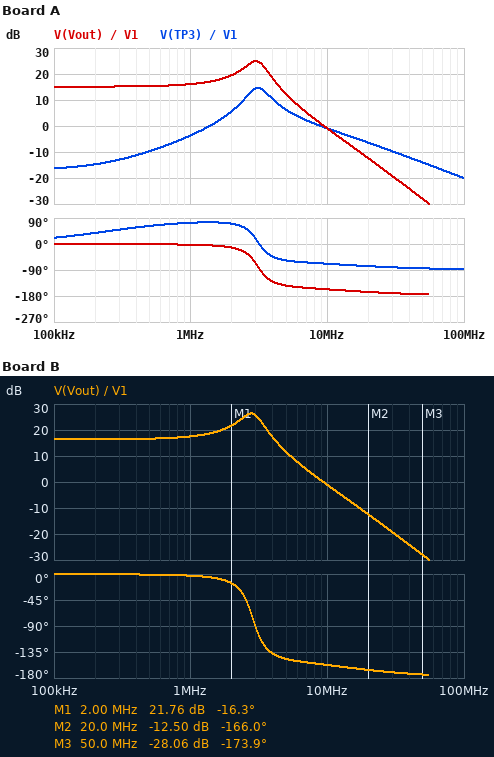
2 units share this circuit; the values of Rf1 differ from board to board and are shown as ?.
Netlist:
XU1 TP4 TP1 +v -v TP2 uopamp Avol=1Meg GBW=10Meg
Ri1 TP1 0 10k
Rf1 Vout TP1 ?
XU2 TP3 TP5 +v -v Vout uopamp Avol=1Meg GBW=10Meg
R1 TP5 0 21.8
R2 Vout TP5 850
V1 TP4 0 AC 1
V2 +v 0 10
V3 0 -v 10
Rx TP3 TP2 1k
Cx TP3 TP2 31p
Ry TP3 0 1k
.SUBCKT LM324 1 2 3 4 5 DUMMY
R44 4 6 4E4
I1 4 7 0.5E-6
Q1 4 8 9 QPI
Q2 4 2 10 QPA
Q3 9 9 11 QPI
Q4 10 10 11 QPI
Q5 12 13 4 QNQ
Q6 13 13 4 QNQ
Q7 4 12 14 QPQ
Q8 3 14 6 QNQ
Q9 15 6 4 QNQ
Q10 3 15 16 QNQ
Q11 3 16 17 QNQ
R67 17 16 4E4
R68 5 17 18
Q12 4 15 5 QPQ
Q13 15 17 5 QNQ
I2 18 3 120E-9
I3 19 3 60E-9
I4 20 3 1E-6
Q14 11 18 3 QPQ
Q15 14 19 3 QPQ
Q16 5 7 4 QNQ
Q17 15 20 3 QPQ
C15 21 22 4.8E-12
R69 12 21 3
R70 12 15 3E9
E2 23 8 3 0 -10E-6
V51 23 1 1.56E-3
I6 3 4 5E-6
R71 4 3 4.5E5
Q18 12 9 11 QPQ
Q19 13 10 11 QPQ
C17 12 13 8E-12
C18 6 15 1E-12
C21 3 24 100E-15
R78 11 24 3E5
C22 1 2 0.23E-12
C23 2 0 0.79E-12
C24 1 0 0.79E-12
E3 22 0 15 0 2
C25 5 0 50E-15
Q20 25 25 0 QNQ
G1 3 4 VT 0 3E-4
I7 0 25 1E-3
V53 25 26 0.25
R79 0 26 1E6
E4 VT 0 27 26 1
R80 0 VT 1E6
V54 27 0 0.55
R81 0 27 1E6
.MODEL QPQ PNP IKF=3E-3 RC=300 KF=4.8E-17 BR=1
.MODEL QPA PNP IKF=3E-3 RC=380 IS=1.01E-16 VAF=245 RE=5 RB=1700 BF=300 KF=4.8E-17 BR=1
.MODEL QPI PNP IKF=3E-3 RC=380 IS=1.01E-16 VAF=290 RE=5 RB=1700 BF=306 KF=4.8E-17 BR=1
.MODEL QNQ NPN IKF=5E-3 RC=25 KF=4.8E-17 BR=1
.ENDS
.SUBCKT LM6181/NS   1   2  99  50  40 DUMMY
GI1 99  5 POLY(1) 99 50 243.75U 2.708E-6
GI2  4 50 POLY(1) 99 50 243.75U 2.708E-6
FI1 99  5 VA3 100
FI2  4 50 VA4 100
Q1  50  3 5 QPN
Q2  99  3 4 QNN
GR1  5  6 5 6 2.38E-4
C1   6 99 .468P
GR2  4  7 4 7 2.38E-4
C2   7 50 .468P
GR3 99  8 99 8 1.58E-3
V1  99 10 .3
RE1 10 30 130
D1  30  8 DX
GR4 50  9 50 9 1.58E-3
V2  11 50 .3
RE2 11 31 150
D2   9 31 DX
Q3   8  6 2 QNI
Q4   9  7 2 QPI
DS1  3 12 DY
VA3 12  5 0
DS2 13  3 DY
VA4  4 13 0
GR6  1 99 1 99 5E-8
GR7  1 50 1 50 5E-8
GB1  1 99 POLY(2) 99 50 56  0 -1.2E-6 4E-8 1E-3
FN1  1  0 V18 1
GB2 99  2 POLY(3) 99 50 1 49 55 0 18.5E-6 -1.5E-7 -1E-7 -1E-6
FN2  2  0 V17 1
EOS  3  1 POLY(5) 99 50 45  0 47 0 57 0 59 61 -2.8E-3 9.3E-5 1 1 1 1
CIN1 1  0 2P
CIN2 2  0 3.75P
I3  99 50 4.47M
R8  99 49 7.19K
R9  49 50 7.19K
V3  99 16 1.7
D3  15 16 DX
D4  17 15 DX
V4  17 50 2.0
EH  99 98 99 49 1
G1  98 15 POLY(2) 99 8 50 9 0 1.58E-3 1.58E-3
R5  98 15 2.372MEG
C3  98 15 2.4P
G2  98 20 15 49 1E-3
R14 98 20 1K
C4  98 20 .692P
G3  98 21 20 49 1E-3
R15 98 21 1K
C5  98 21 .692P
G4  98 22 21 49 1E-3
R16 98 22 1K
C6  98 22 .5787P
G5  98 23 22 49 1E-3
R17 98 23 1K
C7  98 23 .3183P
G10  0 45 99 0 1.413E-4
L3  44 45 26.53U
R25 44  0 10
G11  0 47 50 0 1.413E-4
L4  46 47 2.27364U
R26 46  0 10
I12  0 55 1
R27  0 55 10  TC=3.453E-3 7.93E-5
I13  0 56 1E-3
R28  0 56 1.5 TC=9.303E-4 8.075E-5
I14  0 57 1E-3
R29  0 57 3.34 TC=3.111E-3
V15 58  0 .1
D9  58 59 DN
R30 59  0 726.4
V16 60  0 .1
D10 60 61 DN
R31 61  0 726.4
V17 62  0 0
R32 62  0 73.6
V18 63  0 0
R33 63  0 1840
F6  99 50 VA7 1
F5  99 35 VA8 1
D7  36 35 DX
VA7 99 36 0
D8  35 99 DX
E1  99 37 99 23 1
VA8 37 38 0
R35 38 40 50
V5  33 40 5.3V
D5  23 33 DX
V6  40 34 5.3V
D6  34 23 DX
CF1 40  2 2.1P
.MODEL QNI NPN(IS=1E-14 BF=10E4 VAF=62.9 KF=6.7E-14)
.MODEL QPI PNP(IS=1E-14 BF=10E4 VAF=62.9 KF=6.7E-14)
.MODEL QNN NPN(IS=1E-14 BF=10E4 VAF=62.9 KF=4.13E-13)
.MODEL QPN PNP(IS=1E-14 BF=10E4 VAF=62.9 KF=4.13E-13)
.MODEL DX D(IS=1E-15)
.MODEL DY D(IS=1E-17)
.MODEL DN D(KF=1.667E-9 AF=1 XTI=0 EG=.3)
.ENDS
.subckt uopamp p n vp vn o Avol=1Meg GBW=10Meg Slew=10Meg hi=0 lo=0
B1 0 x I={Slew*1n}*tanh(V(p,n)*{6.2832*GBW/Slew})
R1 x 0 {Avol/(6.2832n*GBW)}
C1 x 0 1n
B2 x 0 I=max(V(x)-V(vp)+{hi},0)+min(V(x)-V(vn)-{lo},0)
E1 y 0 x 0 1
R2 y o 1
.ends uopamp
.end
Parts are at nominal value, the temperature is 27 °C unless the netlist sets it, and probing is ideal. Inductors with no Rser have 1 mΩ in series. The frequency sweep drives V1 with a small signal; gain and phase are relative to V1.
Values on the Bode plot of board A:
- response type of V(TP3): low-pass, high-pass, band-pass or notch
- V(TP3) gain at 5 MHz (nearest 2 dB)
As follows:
band-pass
6 dB
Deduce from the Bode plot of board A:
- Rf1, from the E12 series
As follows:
47 kΩ
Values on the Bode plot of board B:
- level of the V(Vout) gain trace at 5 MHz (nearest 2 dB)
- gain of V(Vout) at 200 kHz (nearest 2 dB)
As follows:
12 dB
16 dB
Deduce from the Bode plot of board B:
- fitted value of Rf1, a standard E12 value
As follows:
56 kΩ
